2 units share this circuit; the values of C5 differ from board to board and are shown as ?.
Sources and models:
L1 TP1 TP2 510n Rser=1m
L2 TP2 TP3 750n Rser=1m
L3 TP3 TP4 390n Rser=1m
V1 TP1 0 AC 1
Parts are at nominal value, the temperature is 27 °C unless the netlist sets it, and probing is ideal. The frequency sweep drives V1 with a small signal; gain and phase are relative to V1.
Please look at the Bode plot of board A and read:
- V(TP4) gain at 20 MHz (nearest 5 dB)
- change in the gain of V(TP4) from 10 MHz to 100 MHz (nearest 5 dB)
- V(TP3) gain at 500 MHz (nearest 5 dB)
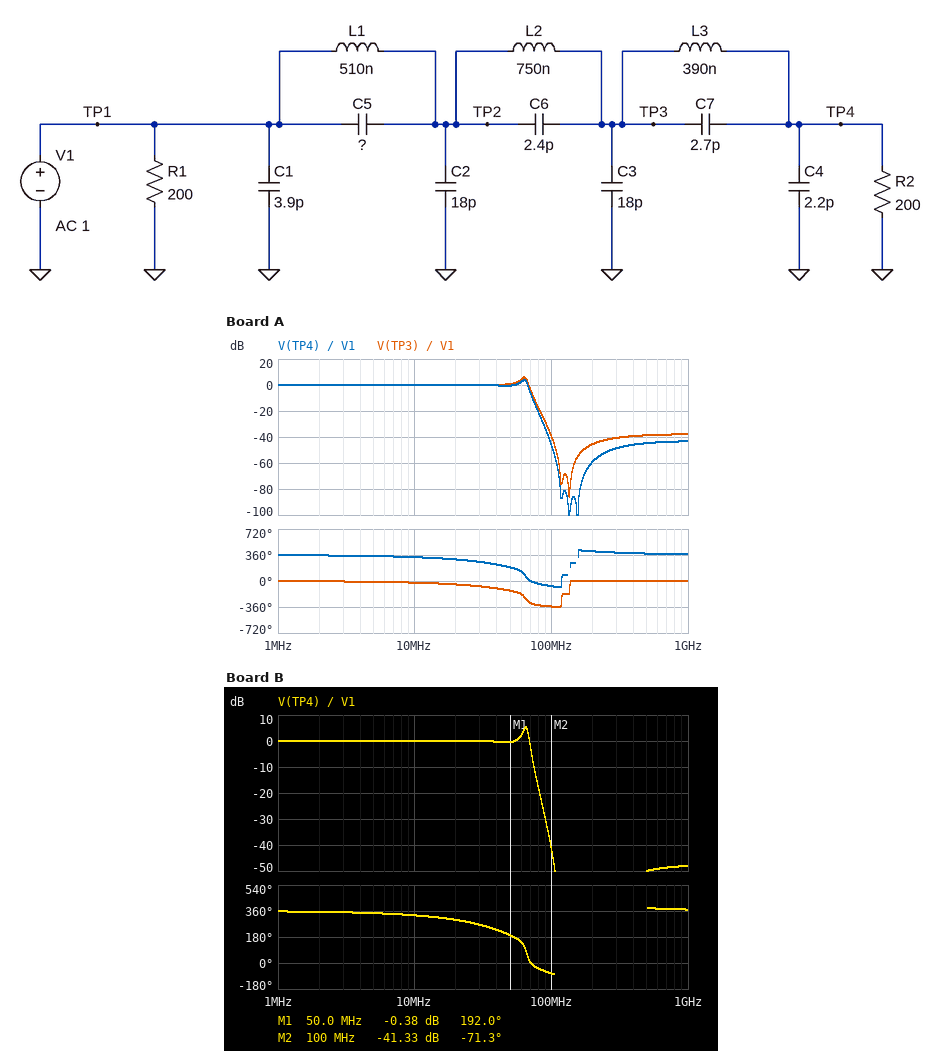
0 dB
-45 dB
-40 dB
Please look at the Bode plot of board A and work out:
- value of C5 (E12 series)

2.7 pF
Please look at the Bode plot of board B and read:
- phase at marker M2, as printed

-71.3 deg
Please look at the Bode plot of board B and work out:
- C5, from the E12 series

1.5 pF
